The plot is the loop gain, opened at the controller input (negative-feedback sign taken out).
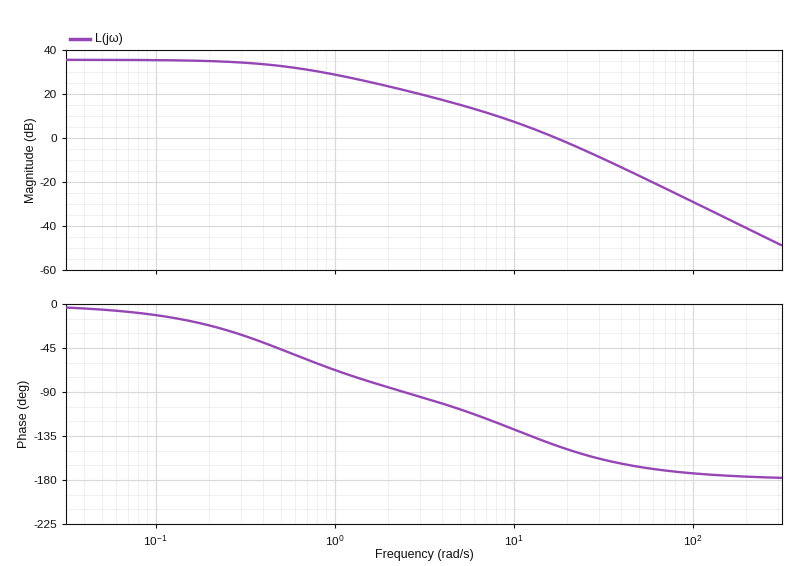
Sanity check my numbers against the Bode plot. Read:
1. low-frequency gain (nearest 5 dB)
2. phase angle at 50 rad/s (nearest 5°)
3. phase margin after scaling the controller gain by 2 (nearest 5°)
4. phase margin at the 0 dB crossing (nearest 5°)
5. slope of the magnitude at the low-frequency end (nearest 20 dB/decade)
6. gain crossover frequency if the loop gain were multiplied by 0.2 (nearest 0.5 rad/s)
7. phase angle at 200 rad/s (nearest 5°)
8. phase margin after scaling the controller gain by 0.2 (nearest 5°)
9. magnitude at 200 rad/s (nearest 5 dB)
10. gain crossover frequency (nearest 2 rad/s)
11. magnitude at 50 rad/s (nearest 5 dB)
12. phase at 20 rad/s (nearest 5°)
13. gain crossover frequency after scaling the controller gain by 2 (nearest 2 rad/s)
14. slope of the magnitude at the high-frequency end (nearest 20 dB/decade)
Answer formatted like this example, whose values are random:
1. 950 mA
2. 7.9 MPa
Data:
1. 35 dB
2. -165°
3. 25°
4. 35°
5. 0 dB/decade
6. 5.5 rad/s
7. -175°
8. 70°
9. -40 dB
10. 18 rad/s
11. -15 dB
12. -150°
13. 26 rad/s
14. -40 dB/decade
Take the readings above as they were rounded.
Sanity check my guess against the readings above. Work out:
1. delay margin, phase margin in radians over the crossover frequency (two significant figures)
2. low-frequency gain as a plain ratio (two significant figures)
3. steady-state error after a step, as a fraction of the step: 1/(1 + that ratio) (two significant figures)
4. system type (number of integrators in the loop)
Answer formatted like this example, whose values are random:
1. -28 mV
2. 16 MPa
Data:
1. 0.034 s
2. 56
3. 0.018
4. 0
